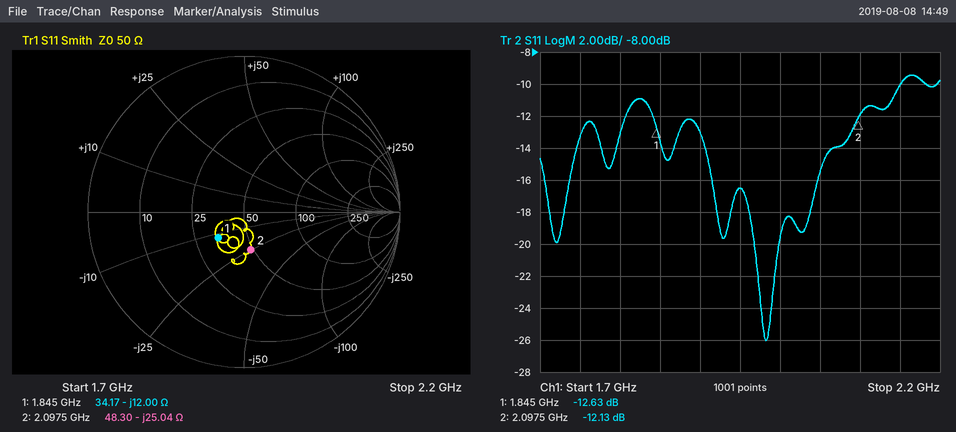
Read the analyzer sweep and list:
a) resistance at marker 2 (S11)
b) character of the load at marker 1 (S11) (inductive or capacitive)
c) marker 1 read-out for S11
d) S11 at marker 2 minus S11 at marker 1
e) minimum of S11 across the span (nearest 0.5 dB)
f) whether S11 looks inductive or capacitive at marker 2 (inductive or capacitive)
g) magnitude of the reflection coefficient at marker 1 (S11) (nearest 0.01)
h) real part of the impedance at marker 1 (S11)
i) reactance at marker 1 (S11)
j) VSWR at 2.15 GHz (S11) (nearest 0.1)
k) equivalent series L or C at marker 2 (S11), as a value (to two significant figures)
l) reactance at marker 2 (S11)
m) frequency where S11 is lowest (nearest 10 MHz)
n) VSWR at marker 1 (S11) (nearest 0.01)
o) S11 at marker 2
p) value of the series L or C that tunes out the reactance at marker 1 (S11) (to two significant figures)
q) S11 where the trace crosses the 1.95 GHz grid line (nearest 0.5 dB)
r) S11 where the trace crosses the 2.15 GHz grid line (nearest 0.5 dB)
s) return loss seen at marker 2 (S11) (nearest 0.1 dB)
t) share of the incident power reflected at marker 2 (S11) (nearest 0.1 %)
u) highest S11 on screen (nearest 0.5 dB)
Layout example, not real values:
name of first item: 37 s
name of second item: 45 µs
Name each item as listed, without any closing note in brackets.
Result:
resistance at marker 2: 48.30 Ω
character of the load at marker 1 (S11): capacitive
marker 1 read-out for S11: -12.63 dB
S11 at marker 2 minus S11 at marker 1: 0.50 dB
minimum of S11 across the span: -26.0 dB
whether S11 looks inductive or capacitive at marker 2: capacitive
magnitude of the reflection coefficient at marker 1 (S11): 0.23
real part of the impedance at marker 1: 34.17 Ω
reactance at marker 1: -12.00 Ω
VSWR at 2.15 GHz (S11): 1.9
equivalent series L or C at marker 2 (S11), as a value: 3.0 pF
reactance at marker 2: -25.04 Ω
frequency where S11 is lowest: 1.98 GHz
VSWR at marker 1 (S11): 1.61
S11 at marker 2: -12.13 dB
value of the series L or C that tunes out the reactance at marker 1 (S11): 1.0 nH
S11 where the trace crosses the 1.95 GHz grid line: -16.5 dB
S11 where the trace crosses the 2.15 GHz grid line: -10.0 dB
return loss seen at marker 2 (S11): 12.1 dB
share of the incident power reflected at marker 2 (S11): 6.1 %
highest S11 on screen: -9.5 dB
